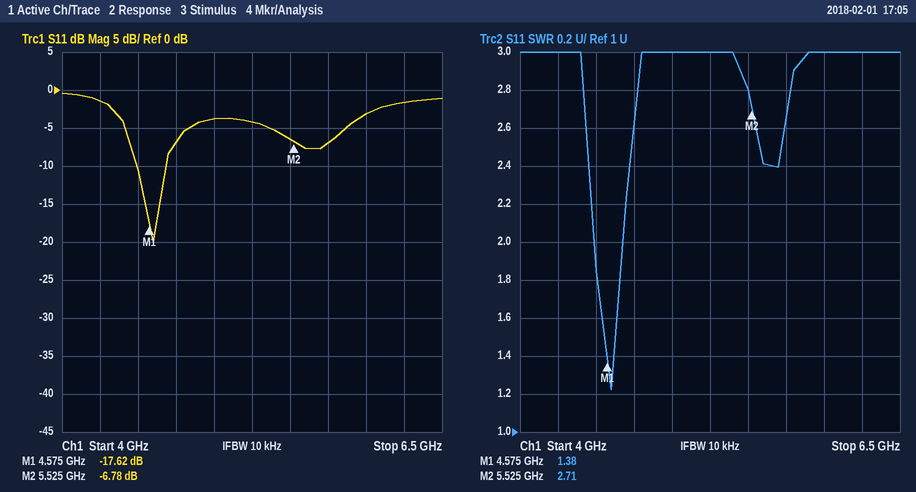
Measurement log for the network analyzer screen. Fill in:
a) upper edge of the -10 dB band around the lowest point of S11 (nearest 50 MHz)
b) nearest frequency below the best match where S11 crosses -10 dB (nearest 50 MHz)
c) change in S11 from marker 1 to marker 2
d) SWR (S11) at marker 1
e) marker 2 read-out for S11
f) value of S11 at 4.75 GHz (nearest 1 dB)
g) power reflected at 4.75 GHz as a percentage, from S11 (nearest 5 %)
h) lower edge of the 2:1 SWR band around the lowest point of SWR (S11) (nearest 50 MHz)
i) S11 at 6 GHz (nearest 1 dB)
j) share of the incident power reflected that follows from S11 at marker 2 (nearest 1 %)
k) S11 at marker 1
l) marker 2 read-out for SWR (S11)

4.70 GHz
4.50 GHz
10.84 dB
1.38
-6.78 dB
-7 dB
20 %
4.50 GHz
-3 dB
21 %
-17.62 dB
2.71
